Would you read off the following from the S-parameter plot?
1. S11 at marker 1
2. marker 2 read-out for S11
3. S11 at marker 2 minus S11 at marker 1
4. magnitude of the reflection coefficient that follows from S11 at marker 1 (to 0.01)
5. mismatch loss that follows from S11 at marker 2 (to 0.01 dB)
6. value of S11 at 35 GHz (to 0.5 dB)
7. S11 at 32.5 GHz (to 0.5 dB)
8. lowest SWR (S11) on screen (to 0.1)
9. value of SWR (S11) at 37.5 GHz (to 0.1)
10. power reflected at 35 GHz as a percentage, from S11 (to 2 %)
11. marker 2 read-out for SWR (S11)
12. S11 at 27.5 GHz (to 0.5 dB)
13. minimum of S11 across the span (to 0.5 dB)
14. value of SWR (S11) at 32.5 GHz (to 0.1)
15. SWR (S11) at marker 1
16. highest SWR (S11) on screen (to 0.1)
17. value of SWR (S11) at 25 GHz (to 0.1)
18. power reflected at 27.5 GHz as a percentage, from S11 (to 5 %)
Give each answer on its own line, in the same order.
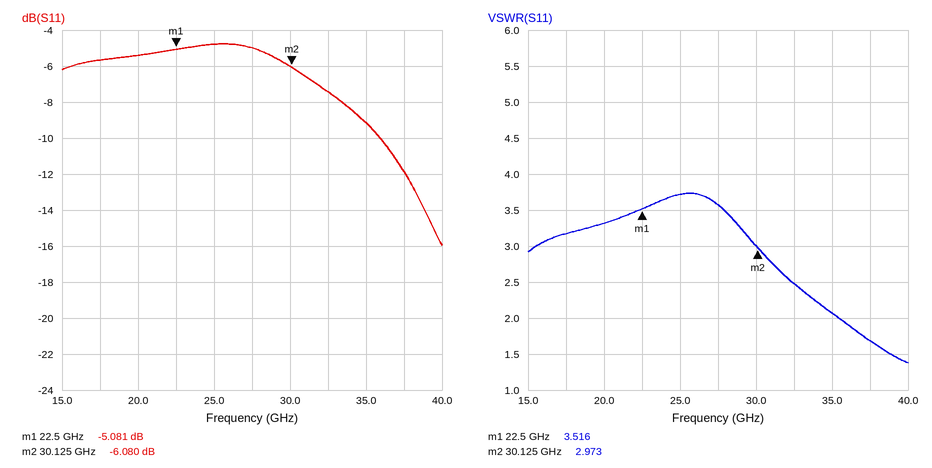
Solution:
-5.081 dB
-6.080 dB
-0.999 dB
0.56
1.23 dB
-9.0 dB
-7.5 dB
1.4
1.7
12 %
2.973
-5.0 dB
-16.0 dB
2.5
3.516
3.7
3.7
30 %
